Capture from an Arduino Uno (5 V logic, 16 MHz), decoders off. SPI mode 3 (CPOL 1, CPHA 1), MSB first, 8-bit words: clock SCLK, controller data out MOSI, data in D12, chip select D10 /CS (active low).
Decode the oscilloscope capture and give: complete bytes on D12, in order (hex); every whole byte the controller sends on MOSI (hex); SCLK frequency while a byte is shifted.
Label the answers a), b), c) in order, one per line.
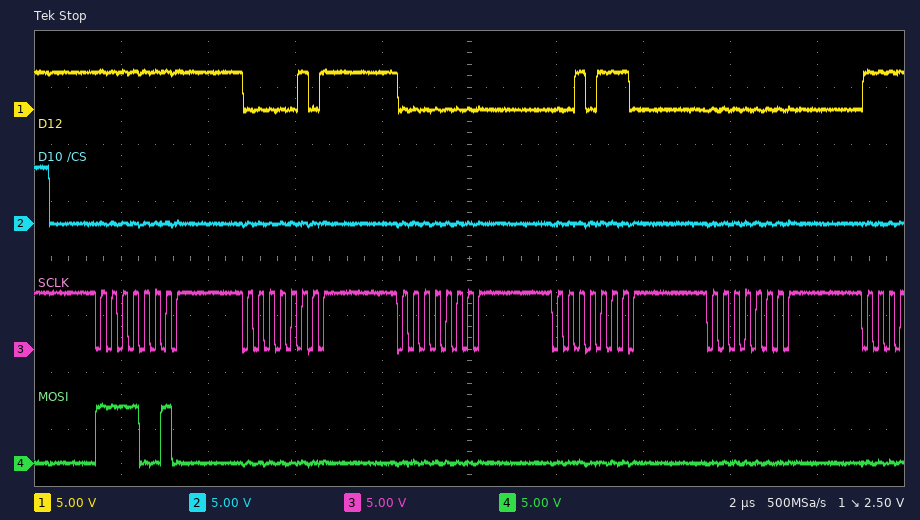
a) FF 05 00 2E 00
b) F2 00 00 00 00
c) 4 MHz
